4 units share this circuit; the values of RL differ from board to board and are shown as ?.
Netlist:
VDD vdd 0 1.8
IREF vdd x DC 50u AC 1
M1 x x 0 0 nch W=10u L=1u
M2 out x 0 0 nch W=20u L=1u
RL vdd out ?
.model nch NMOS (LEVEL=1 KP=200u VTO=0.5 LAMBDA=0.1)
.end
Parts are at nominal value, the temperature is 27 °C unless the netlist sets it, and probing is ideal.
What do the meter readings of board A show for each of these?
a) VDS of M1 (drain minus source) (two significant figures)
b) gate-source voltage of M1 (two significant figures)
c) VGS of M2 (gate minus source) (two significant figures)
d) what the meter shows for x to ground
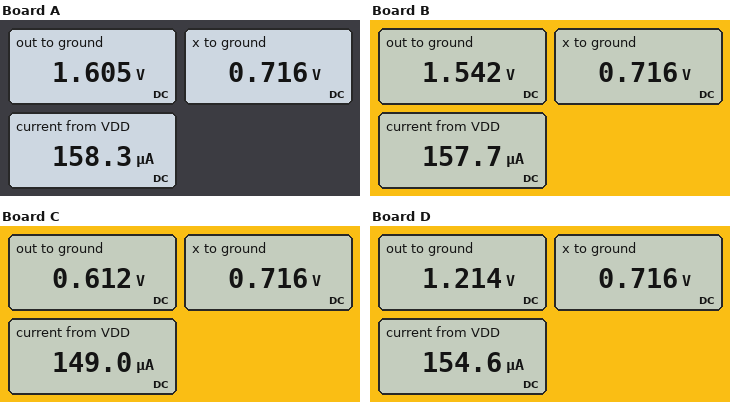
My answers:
720 mV
720 mV
720 mV
0.716 V
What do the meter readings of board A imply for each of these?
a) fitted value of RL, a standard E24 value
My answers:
1.8 kΩ
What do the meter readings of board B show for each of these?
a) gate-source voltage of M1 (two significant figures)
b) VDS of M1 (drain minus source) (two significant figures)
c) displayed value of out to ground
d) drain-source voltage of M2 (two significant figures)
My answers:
720 mV
720 mV
1.542 V
1.5 V
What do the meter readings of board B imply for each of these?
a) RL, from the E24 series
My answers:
2.4 kΩ
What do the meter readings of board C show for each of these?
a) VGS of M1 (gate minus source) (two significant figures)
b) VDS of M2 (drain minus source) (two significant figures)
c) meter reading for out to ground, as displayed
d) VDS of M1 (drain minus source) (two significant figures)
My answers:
720 mV
610 mV
0.612 V
720 mV
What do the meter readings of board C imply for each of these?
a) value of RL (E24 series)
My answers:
12 kΩ
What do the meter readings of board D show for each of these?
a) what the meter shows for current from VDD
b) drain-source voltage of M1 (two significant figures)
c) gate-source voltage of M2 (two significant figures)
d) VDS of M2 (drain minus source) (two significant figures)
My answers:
154.6 µA
720 mV
720 mV
1.2 V
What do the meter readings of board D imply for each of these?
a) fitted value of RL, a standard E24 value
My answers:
5.6 kΩ
